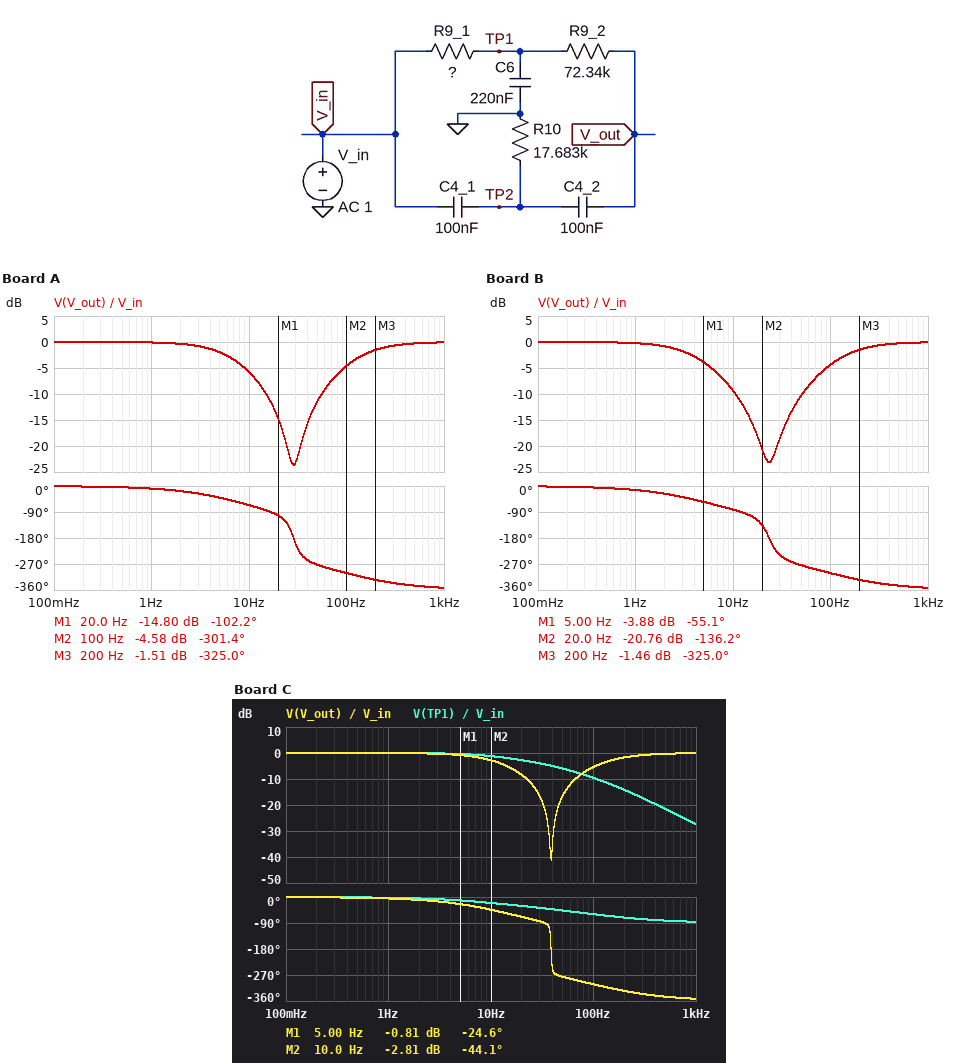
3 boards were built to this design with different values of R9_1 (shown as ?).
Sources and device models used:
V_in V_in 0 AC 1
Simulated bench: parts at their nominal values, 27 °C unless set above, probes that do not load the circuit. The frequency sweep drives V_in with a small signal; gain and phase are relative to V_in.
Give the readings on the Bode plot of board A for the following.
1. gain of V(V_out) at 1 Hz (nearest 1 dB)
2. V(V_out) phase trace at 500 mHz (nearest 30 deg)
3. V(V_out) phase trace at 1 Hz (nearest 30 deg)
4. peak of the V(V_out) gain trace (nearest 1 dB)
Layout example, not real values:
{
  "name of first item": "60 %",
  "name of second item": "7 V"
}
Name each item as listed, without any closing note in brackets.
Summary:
{
  "gain of V(V_out) at 1 Hz": "0 dB",
  "V(V_out) phase trace at 500 mHz": "0 deg",
  "V(V_out) phase trace at 1 Hz": "0 deg",
  "peak of the V(V_out) gain trace": "0 dB"
}
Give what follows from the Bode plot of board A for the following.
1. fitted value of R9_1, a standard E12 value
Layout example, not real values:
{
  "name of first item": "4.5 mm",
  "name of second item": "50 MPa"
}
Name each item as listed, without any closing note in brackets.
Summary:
{
  "fitted value of R9_1, a standard E12 value": "56 kΩ"
}
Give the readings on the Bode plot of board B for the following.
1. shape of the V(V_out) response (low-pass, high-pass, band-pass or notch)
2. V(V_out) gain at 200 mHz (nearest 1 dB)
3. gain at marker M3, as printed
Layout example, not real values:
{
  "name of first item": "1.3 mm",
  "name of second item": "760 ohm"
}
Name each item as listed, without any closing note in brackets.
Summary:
{
  "shape of the V(V_out) response": "notch",
  "V(V_out) gain at 200 mHz": "0 dB",
  "gain at marker M3, as printed": "-1.46 dB"
}
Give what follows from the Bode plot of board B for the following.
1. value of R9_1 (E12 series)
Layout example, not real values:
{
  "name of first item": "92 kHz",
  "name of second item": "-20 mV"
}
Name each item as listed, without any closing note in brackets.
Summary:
{
  "value of R9_1": "100 kΩ"
}
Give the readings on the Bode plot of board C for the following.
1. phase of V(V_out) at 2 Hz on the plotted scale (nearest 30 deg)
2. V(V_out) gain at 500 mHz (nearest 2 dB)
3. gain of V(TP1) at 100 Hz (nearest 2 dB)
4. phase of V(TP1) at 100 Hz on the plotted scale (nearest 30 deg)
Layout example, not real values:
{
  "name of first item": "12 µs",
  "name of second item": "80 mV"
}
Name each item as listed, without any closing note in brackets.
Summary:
{
  "phase of V(V_out) at 2 Hz on the plotted scale": "0 deg",
  "V(V_out) gain at 500 mHz": "0 dB",
  "gain of V(TP1) at 100 Hz": "-10 dB",
  "phase of V(TP1) at 100 Hz on the plotted scale": "-60 deg"
}
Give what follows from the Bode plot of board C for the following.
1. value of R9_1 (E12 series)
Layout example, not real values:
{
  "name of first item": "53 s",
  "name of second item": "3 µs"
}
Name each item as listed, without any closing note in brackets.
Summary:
{
  "value of R9_1": "22 kΩ"
}
